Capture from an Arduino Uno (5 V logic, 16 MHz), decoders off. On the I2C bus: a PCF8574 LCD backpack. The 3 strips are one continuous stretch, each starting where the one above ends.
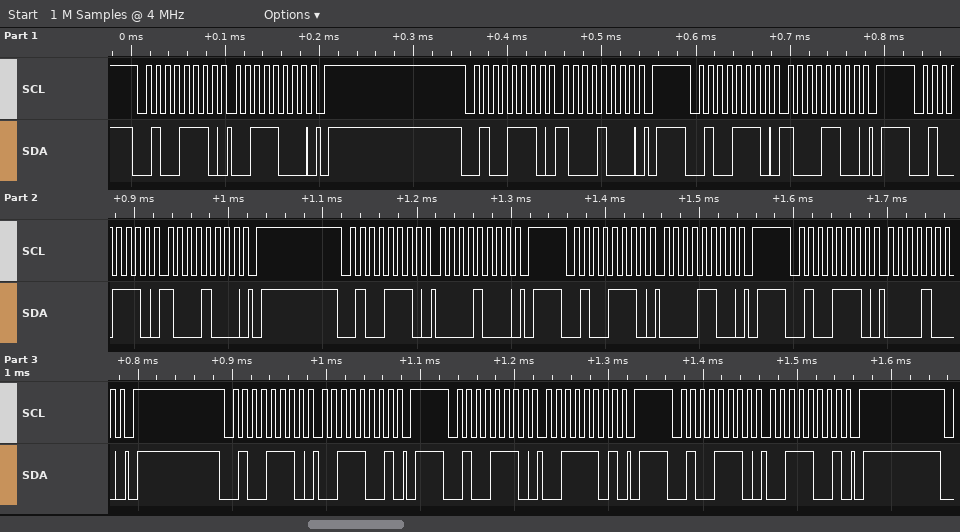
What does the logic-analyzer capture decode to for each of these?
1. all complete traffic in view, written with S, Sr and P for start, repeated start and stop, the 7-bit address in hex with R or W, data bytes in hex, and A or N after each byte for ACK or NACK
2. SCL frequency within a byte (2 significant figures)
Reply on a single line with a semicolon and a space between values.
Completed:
S 27W A 38 A P S 27W A 88 A P S 27W A 8C A P S 27W A 88 A P S 27W A 08 A P S 27W A 0C A P S 27W A 08 A P S 27W A 39 A P S 27W A 3D A P S 27W A 39 A P; 100 kHz
